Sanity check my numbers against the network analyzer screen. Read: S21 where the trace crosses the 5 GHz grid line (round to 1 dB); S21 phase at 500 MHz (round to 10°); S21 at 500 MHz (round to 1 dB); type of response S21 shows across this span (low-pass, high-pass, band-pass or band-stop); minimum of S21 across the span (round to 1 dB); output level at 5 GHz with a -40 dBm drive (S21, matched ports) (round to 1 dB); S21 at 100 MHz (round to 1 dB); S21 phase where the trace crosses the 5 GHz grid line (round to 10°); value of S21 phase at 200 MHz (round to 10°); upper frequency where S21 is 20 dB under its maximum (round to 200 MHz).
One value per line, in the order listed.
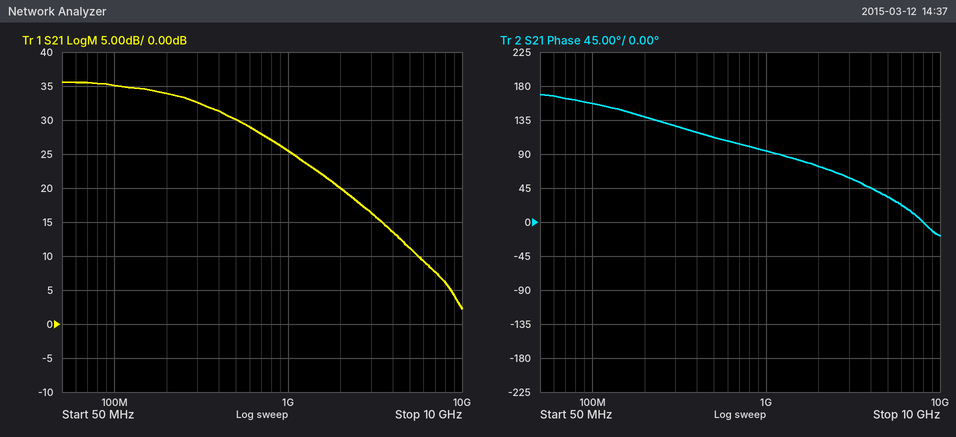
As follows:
11 dB
110°
30 dB
low-pass
2 dB
-29 dBm
35 dB
30°
140°
3.2 GHz
